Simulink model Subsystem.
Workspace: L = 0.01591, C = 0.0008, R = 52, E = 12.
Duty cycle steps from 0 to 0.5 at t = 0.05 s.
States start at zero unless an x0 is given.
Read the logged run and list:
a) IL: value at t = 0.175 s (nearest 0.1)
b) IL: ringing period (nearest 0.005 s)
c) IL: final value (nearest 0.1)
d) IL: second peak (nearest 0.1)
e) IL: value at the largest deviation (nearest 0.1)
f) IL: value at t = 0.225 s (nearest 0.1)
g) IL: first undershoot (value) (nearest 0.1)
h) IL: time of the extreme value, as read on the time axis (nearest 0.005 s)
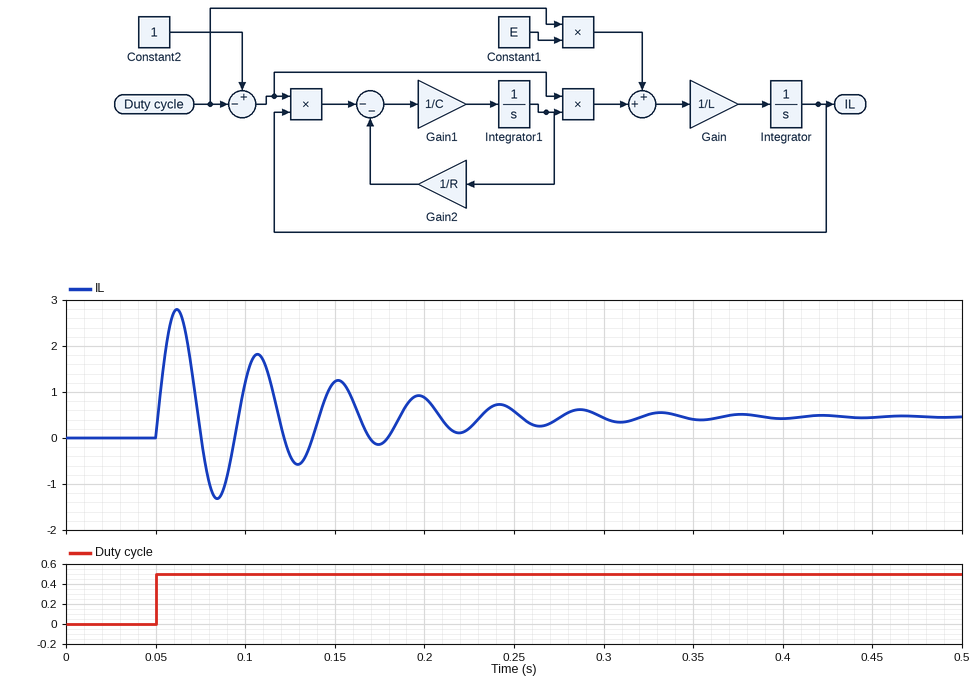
-0.1
0.045 s
0.5
1.8
2.8
0.2
-1.3
0.060 s
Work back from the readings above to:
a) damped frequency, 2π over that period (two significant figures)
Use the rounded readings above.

140 rad/s
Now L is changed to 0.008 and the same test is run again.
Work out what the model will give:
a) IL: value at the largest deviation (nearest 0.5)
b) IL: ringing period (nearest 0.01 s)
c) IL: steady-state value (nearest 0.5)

4.0
0.03 s
0.5
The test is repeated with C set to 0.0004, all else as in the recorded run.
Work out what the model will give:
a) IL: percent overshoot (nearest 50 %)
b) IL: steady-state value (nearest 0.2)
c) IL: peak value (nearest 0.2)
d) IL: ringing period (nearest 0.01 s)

350 %
0.4
2.0
0.03 s
